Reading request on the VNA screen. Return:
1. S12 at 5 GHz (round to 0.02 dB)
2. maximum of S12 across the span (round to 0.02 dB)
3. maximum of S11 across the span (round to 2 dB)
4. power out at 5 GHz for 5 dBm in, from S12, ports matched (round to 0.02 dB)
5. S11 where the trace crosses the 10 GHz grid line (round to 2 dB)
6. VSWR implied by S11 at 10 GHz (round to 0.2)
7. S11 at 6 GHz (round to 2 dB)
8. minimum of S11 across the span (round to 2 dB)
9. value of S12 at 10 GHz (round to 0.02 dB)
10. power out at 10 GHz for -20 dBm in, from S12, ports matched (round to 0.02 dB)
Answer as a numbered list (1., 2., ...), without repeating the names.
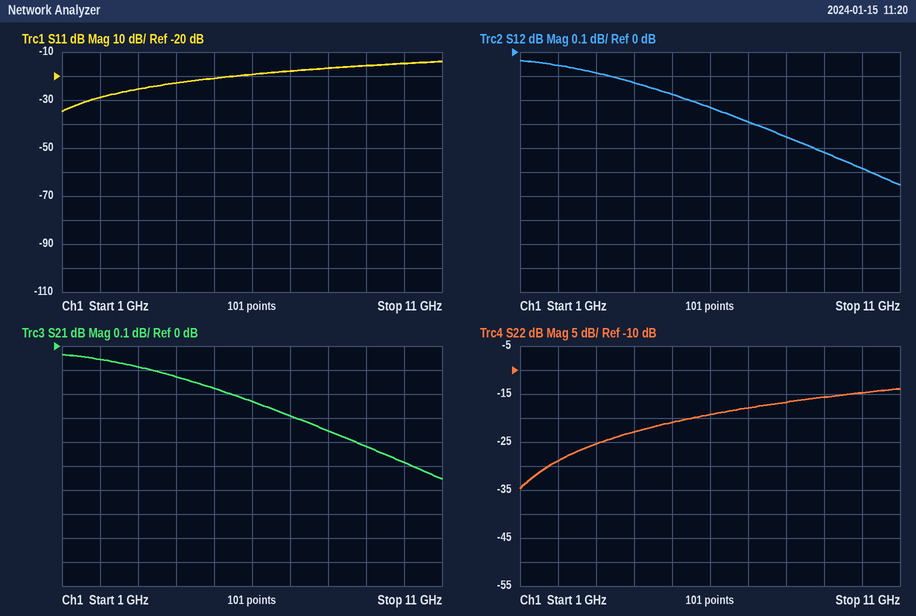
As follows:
1. -0.18 dB
2. -0.04 dB
3. -14 dB
4. 4.82 dBm
5. -14 dB
6. 1.4
7. -20 dB
8. -34 dB
9. -0.48 dB
10. -20.48 dBm
